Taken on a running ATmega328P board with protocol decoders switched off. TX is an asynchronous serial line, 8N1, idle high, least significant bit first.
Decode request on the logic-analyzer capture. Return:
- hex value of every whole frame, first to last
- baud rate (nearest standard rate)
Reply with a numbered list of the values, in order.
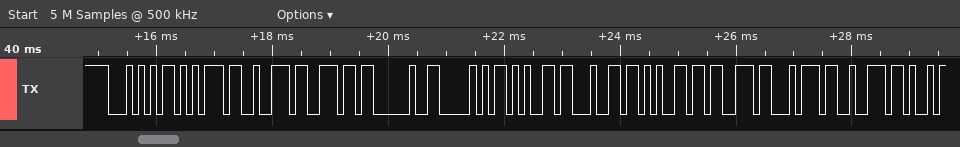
1. 0x54 0x75 0x72 0x6E 0x20 0x50 0x65 0x64 0x65 0x73 0x74 0x72
2. 9600 baud
